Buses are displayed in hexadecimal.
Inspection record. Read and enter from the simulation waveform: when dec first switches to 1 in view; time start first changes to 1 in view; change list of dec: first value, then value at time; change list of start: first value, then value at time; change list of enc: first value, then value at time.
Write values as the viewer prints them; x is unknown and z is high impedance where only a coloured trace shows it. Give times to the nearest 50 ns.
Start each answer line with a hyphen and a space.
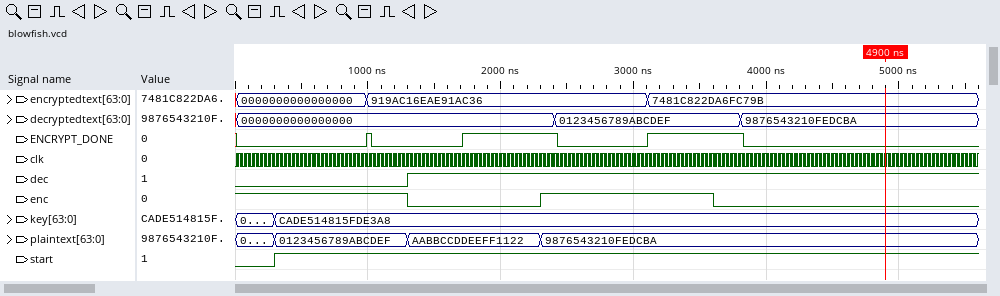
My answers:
- 1300 ns
- 300 ns
- 0, 1 at 1300 ns
- 0, 1 at 300 ns
- 1, 0 at 1300 ns, 1 at 2300 ns, 0 at 3600 ns
